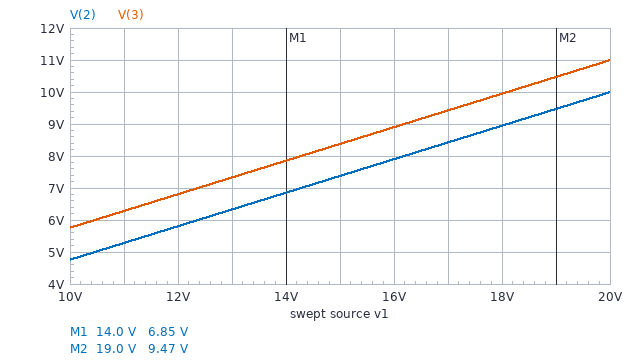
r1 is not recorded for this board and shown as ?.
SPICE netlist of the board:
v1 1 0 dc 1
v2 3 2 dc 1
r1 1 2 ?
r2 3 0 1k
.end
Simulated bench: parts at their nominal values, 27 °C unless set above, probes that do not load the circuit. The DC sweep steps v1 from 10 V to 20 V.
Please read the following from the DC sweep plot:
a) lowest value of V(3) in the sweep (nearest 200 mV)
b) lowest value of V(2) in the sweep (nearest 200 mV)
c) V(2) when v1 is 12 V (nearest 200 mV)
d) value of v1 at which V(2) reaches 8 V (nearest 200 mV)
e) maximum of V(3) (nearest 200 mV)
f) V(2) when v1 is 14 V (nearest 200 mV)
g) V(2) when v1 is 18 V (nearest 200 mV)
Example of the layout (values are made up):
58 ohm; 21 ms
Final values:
5.8 V; 4.8 V; 5.8 V; 16.2 V; 11.0 V; 6.8 V; 9.0 V
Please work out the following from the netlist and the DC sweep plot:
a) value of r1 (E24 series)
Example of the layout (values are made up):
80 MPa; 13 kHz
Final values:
910 Ω
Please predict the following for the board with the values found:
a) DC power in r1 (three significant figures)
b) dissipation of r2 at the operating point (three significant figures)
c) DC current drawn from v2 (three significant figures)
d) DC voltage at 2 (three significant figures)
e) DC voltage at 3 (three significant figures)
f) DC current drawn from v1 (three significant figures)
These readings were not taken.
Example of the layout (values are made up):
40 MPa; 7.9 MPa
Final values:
998 µW; 1.10 mW; 1.05 mA; 47.1 mV; 1.05 V; 1.05 mA
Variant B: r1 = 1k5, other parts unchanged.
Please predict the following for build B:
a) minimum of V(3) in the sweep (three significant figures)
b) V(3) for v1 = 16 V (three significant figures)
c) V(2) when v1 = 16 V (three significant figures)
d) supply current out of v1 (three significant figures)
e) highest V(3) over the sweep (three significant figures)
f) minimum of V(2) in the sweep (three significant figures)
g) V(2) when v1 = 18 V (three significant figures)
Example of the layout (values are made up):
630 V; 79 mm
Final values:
4.40 V; 6.80 V; 5.80 V; 800 µA; 8.40 V; 3.40 V; 6.60 V
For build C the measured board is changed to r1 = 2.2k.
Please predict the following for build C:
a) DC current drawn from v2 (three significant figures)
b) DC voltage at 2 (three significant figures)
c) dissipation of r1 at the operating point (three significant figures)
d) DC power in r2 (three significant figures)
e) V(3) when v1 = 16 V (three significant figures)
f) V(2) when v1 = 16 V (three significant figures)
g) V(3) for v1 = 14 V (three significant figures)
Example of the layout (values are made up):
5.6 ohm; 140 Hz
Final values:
625 µA; -375 mV; 859 µW; 391 µW; 5.31 V; 4.31 V; 4.69 V
